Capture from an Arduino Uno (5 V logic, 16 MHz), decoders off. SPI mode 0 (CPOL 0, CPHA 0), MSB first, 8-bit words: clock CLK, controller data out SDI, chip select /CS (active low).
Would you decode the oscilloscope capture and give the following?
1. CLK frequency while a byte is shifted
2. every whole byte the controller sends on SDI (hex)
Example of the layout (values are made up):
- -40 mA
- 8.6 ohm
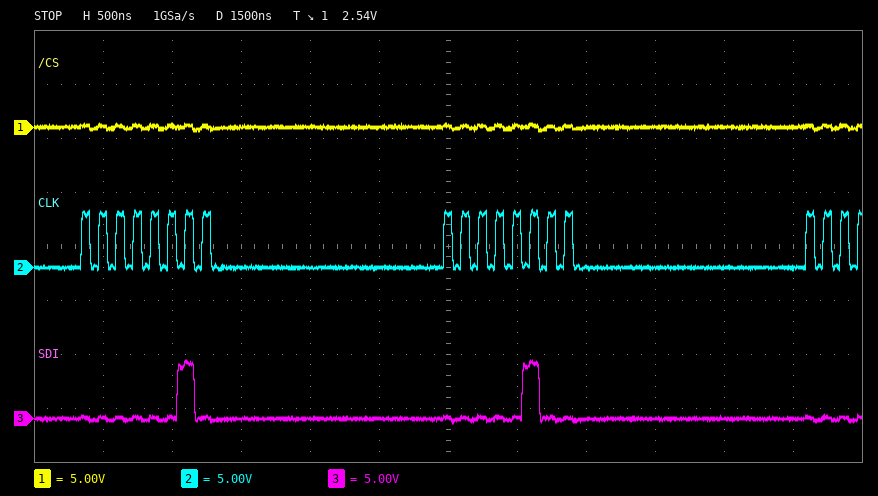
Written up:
- 8 MHz
- 0x02 0x04
